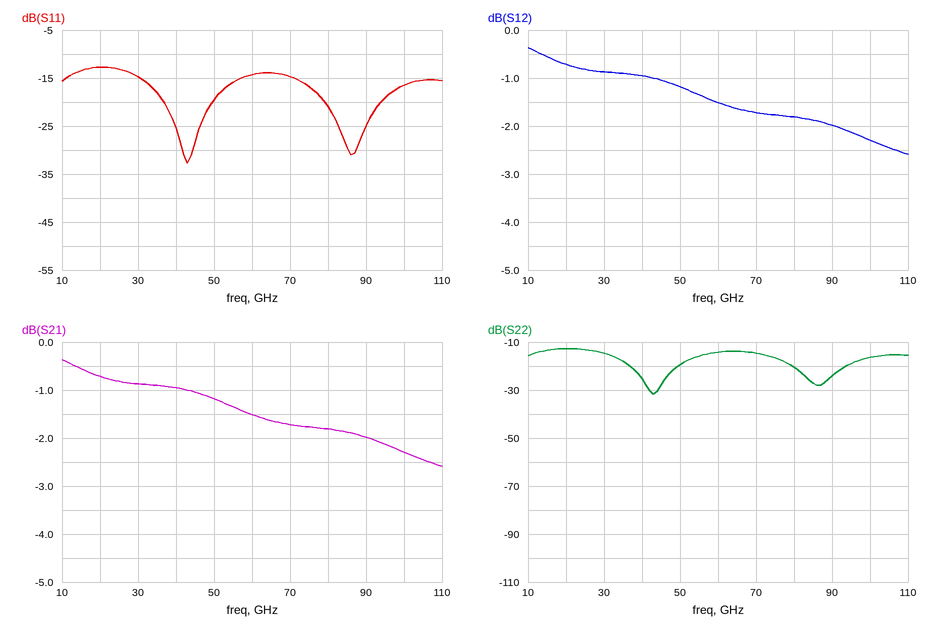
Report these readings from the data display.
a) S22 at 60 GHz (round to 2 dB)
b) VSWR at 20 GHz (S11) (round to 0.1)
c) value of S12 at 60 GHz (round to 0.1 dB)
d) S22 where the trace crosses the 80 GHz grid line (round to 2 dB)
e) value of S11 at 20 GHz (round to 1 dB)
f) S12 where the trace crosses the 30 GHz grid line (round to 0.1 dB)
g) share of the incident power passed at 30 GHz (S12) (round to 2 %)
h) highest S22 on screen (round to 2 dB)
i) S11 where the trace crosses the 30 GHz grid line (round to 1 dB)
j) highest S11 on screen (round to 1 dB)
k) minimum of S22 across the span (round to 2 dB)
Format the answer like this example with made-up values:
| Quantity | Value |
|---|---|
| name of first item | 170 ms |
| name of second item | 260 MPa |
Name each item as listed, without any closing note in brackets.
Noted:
| Quantity | Value |
|---|---|
| S22 at 60 GHz | -14 dB |
| VSWR at 20 GHz (S11) | 1.6 |
| value of S12 at 60 GHz | -1.5 dB |
| S22 where the trace crosses the 80 GHz grid line | -20 dB |
| value of S11 at 20 GHz | -13 dB |
| S12 where the trace crosses the 30 GHz grid line | -0.9 dB |
| share of the incident power passed at 30 GHz (S12) | 82 % |
| highest S22 on screen | -12 dB |
| S11 where the trace crosses the 30 GHz grid line | -15 dB |
| highest S11 on screen | -13 dB |
| minimum of S22 across the span | -32 dB |
